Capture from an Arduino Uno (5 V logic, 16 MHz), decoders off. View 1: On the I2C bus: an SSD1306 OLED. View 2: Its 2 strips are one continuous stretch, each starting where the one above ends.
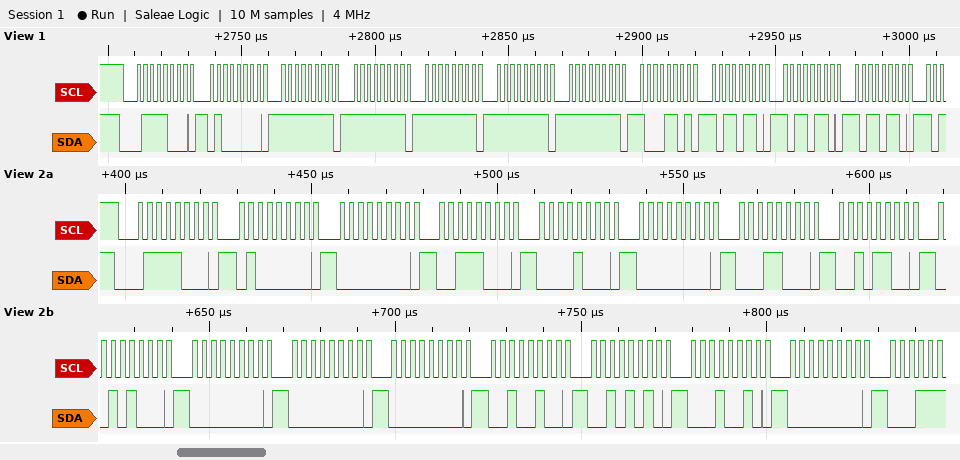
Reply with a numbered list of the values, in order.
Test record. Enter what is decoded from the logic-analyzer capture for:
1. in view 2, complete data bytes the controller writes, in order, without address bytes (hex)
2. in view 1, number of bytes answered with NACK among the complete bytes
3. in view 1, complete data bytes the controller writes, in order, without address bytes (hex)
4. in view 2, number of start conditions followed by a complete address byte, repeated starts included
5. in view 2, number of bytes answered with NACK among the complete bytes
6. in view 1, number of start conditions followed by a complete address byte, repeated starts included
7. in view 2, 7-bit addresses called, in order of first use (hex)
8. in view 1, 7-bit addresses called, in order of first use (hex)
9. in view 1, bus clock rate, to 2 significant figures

1. 40 00 38 08 00 18 2C 28 00 00 00 24 2A 12 00
2. 0
3. 40 FF FF FF FF FF 8D B6 B6 B6
4. 1
5. 0
6. 1
7. 0x3C
8. 0x3C
9. 400 kHz
